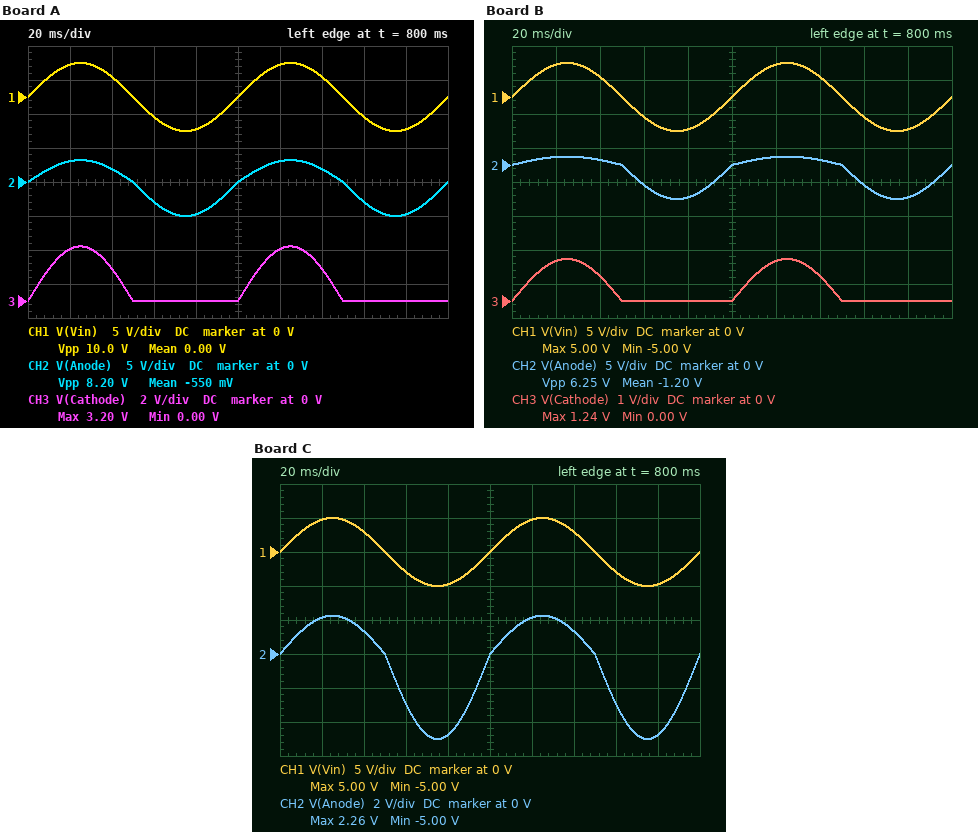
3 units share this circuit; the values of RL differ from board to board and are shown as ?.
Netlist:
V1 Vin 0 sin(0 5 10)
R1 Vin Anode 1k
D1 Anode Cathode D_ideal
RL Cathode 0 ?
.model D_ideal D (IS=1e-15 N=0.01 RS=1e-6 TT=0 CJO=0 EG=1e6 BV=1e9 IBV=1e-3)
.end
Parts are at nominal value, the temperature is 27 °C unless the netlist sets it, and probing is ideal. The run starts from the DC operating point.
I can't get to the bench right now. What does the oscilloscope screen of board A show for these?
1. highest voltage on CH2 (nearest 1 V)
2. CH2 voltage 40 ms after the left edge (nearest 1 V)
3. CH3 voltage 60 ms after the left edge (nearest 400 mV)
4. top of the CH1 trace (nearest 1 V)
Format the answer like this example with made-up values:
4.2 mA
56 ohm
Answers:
3 V
2 V
0 V
5 V
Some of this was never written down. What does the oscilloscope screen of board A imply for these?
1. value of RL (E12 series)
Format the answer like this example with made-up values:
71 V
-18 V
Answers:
1.8 kΩ
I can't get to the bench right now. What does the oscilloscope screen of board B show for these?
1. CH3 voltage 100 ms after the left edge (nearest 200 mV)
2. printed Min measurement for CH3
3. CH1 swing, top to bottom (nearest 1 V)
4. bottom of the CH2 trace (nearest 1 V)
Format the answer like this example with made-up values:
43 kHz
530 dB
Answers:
0 V
0.00 V
10 V
-5 V
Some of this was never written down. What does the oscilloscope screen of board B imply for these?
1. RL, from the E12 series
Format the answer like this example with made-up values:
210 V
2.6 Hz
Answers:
330 Ω
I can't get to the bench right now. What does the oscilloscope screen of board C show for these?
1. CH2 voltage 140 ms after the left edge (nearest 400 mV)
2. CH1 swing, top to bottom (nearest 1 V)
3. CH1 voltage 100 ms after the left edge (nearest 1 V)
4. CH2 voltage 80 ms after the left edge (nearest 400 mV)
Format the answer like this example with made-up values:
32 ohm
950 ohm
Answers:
1.2 V
10 V
0 V
-4.8 V
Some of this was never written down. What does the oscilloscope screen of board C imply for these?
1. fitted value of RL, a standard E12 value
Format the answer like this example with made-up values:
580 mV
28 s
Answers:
820 Ω
